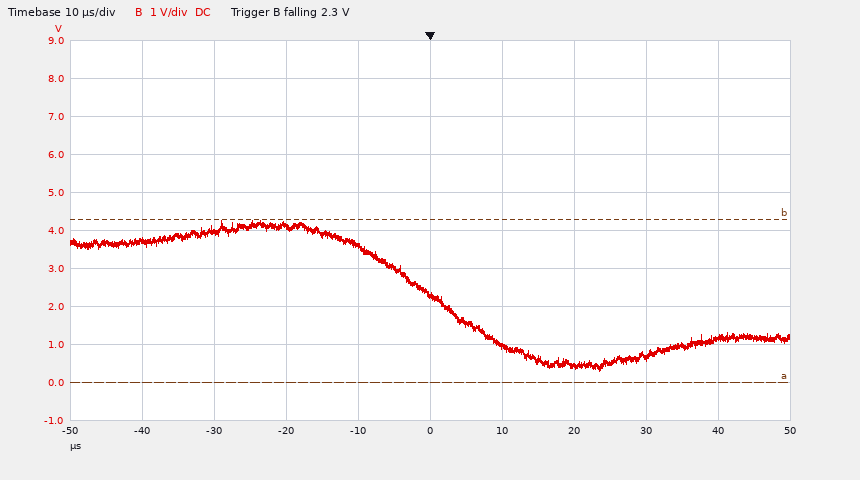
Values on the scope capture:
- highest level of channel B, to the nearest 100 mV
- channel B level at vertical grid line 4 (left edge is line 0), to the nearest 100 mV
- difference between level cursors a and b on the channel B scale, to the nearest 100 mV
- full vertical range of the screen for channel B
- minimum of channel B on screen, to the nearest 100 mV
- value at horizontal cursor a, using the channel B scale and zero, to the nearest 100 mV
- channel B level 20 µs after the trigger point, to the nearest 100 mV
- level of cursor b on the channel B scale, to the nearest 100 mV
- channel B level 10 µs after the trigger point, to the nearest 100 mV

4.3 V
3.6 V
4.3 V
10 V
300 mV
0.0 V
400 mV
4.3 V
1.0 V
